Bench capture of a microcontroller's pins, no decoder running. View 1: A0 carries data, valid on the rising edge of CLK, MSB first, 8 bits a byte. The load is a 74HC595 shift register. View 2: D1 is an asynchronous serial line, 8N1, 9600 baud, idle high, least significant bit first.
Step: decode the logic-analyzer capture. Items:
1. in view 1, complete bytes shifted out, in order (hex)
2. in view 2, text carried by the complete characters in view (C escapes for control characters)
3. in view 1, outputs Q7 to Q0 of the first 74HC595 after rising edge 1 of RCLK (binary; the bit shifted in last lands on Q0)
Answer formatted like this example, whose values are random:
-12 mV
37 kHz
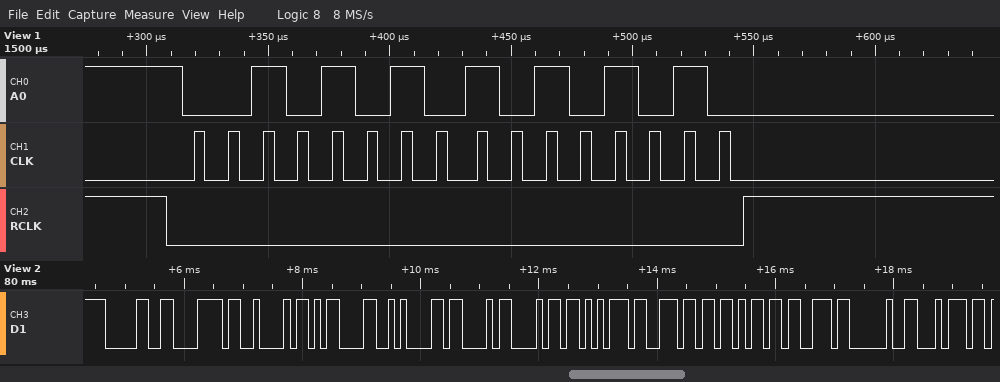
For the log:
2A AA
"0xB\r\nChunks t"
10101010
